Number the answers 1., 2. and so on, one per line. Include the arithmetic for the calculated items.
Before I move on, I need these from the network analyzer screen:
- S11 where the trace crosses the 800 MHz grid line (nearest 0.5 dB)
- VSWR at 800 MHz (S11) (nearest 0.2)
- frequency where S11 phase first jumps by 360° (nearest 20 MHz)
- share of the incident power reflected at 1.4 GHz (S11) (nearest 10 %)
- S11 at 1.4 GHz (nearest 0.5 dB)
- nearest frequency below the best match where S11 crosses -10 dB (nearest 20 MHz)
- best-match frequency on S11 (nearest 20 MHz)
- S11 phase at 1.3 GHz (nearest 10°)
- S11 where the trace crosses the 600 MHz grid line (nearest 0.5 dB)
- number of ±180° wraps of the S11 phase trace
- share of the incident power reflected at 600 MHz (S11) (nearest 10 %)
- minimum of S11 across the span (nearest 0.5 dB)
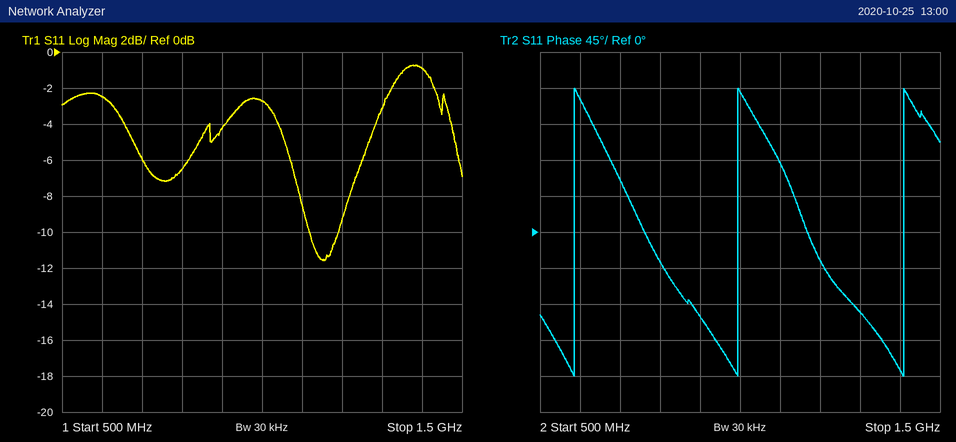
1. -6.5 dB
2. |Γ| = 10^(-6.5/20) = 0.4732; VSWR = (1 + 0.4732)/(1 − 0.4732) ≈ 2.8
3. 580 MHz
4. 10^(-1/10) ≈ 79.4 %, so 80 % to the nearest 10 %
5. -1.0 dB
6. 1.12 GHz
7. 1.16 GHz
8. -100°
9. -2.5 dB
10. 3
11. 10^(-2.5/10) ≈ 56.2 %, so 60 % to the nearest 10 %
12. -11.5 dB
